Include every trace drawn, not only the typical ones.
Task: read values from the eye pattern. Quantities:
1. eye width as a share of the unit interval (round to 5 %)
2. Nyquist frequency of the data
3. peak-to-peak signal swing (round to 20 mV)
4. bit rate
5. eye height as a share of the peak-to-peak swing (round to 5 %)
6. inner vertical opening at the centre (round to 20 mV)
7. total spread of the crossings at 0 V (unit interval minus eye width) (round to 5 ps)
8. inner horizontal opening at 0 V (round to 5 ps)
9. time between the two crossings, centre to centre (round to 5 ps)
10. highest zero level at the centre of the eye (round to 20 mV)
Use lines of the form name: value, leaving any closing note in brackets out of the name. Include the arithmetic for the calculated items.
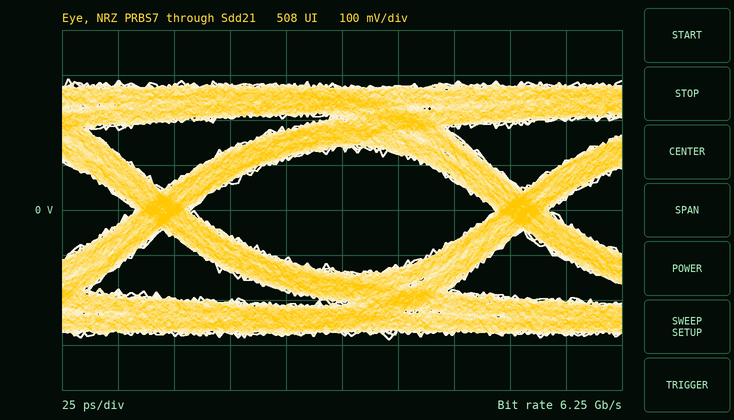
eye width as a share of the unit interval: 135 ps / 160 ps ≈ 84.4 %, so 85 % to the nearest 5 %
Nyquist frequency of the data: 3.125 GHz
peak-to-peak signal swing: 580 mV
bit rate: 6.25 Gb/s
eye height as a share of the peak-to-peak swing: 280 mV / 580 mV ≈ 48.3 %, so 50 % to the nearest 5 %
inner vertical opening at the centre: 280 mV
total spread of the crossings at 0 V (unit interval minus eye width): 25 ps
inner horizontal opening at 0 V: 135 ps
time between the two crossings, centre to centre: 160 ps
highest zero level at the centre of the eye: -140 mV
